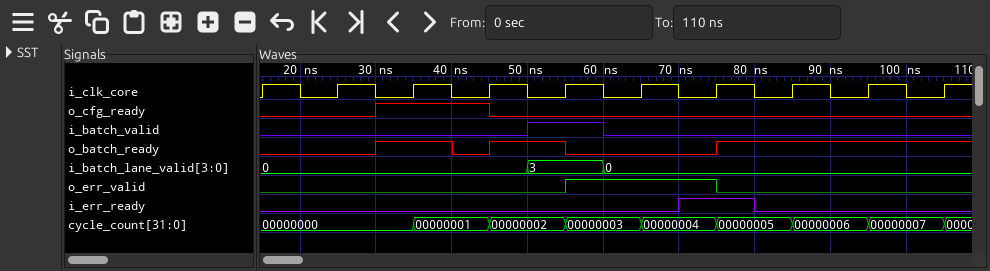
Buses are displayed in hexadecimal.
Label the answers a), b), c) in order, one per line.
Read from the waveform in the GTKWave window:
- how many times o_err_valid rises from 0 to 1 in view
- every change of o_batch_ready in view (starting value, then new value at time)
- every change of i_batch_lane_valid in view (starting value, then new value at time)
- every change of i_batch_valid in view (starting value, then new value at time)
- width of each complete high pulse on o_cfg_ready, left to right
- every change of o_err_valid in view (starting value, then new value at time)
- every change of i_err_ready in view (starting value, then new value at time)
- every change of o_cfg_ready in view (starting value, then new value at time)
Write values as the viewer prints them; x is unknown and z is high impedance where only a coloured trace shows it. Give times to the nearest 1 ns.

a) 1
b) 0, 1 at 30 ns, 0 at 40 ns, 1 at 45 ns, 0 at 55 ns, 1 at 75 ns
c) 0, 3 at 50 ns, 0 at 60 ns
d) 0, 1 at 50 ns, 0 at 60 ns
e) 15 ns
f) 0, 1 at 55 ns, 0 at 75 ns
g) 0, 1 at 70 ns, 0 at 80 ns
h) 0, 1 at 30 ns, 0 at 45 ns
